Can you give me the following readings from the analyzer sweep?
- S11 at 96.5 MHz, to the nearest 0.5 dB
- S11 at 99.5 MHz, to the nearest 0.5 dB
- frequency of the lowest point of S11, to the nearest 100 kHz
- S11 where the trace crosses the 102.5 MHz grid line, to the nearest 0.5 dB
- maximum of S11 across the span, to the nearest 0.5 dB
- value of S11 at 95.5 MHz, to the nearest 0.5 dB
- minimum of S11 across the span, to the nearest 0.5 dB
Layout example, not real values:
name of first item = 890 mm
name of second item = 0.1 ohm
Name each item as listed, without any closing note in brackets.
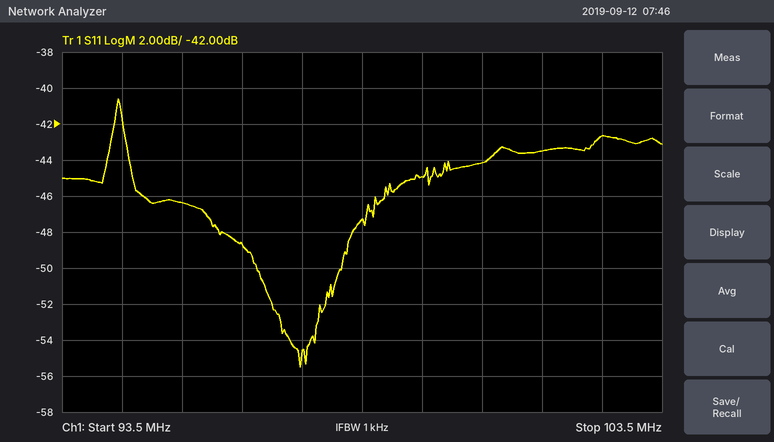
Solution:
S11 at 96.5 MHz, to the nearest 0.5 dB = -48.5 dB
S11 at 99.5 MHz, to the nearest 0.5 dB = -45.0 dB
frequency of the lowest point of S11, to the nearest 100 kHz = 97.5 MHz
S11 where the trace crosses the 102.5 MHz grid line, to the nearest 0.5 dB = -42.5 dB
maximum of S11 across the span, to the nearest 0.5 dB = -40.5 dB
value of S11 at 95.5 MHz, to the nearest 0.5 dB = -46.5 dB
minimum of S11 across the span, to the nearest 0.5 dB = -55.5 dB
